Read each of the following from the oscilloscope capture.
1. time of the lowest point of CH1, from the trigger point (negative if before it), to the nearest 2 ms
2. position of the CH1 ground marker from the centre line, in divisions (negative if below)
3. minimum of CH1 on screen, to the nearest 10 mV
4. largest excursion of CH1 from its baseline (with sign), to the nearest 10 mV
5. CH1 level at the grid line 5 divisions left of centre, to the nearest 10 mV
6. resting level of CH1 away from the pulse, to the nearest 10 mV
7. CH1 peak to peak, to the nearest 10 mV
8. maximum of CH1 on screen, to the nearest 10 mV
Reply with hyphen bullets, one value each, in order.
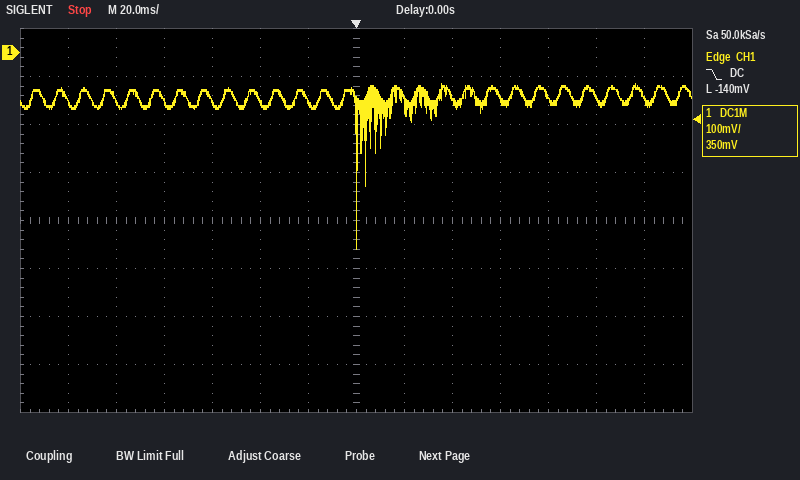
- 0 ms
- +3.5 div
- -410 mV
- -310 mV
- -100 mV
- -100 mV
- 350 mV
- -60 mV
